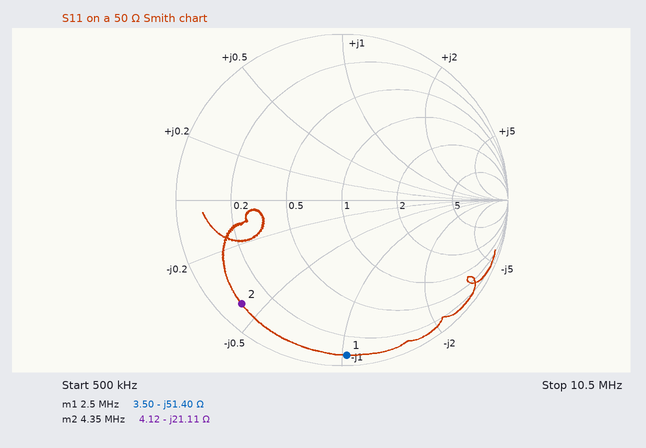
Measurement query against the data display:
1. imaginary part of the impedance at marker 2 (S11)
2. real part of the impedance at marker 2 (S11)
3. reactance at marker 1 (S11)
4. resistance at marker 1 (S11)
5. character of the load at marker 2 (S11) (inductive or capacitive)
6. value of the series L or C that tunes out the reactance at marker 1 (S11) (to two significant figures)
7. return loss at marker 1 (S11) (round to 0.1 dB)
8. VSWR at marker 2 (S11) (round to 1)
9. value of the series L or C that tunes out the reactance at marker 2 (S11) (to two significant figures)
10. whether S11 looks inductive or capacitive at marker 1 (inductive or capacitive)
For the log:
-21.11 Ω
4.12 Ω
-51.40 Ω
3.50 Ω
capacitive
3.3 µH
0.6 dB
14
770 nH
capacitive
